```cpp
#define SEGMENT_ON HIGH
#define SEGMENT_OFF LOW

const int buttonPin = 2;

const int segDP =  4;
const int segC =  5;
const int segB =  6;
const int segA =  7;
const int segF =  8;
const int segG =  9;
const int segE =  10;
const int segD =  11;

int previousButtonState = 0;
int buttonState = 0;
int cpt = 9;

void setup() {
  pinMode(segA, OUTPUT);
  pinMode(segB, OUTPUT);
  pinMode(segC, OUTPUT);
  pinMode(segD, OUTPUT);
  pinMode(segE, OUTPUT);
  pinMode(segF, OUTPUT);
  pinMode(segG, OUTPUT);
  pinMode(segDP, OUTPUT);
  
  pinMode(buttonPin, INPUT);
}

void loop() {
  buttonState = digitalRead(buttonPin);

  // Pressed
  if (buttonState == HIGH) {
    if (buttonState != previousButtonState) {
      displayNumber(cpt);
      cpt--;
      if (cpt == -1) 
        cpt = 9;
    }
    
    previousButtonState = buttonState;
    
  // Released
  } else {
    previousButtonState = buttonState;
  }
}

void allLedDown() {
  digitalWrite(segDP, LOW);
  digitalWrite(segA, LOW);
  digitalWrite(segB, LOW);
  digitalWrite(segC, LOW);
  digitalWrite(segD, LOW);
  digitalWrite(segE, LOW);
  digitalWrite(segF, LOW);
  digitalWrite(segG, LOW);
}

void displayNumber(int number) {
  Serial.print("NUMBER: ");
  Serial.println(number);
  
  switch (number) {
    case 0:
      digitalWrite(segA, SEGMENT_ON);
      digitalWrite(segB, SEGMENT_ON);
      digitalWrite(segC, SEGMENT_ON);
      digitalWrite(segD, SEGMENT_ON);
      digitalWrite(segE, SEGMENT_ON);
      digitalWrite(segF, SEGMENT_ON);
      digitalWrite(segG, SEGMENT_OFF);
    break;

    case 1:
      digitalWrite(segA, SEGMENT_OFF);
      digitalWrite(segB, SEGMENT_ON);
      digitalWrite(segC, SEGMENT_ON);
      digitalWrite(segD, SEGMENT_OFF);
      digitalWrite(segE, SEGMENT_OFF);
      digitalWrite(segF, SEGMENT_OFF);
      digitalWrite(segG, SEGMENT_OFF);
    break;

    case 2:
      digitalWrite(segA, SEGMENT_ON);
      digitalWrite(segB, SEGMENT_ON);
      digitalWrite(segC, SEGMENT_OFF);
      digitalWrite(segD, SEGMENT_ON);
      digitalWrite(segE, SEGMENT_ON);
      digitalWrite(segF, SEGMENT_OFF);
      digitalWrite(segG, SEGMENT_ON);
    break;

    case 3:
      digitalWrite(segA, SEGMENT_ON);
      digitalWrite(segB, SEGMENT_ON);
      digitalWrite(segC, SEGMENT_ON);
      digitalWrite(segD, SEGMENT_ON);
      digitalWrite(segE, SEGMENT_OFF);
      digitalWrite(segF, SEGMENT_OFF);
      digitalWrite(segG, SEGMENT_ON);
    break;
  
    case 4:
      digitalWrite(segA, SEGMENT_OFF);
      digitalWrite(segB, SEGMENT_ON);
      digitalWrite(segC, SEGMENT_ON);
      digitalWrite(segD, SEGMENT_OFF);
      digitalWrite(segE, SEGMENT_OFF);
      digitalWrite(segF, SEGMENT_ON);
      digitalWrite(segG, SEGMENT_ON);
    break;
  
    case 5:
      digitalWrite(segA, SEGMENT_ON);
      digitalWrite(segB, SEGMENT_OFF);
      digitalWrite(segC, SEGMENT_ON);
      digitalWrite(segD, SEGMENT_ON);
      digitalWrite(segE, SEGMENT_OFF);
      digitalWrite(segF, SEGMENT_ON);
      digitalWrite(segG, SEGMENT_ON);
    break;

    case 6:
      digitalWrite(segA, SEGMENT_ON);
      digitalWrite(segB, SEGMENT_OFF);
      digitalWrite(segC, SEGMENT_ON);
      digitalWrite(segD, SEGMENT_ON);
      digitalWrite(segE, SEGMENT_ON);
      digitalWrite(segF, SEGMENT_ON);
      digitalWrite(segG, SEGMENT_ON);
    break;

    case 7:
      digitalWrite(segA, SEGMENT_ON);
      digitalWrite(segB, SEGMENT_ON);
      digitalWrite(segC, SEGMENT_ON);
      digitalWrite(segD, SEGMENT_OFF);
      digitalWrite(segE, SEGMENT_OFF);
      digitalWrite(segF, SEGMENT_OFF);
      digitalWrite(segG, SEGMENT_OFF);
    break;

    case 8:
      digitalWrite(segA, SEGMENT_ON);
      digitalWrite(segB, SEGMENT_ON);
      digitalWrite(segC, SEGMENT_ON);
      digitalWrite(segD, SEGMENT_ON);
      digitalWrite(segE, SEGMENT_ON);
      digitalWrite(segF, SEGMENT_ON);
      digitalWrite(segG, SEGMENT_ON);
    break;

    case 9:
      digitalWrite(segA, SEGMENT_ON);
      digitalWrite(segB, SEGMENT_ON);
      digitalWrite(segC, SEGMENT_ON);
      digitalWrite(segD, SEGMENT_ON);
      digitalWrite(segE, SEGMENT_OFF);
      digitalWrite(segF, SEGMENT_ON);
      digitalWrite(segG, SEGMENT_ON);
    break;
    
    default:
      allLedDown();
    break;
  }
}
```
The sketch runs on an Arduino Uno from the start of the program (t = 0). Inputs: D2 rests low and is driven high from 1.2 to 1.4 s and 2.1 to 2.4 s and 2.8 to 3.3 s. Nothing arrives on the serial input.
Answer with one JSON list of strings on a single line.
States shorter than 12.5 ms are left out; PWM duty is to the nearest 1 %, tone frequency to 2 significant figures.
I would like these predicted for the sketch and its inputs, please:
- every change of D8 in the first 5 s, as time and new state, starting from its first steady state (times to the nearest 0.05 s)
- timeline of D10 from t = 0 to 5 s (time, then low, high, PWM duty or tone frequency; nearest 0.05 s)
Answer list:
["0 s low; 1.2 s high; 2.8 s low", "0 s low; 2.1 s high; 2.8 s low"]
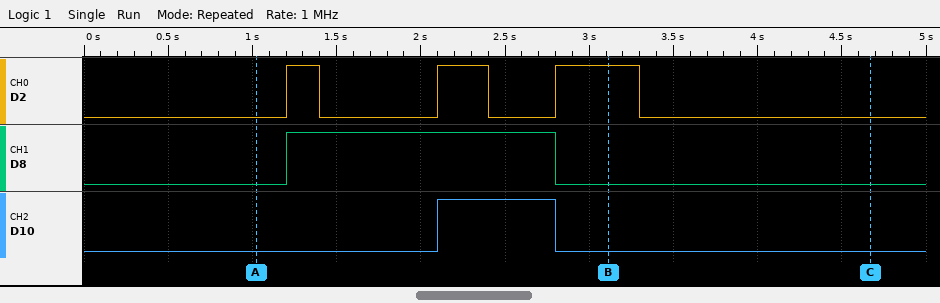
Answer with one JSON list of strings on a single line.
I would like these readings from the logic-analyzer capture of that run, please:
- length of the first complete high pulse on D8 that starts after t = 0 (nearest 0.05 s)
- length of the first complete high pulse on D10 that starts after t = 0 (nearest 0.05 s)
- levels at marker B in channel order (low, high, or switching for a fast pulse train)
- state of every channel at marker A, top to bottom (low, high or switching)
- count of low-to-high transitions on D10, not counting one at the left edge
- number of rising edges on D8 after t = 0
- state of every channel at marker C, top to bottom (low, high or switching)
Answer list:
["1.60 s", "0.70 s", "D2 high, D8 low, D10 low", "D2 low, D8 low, D10 low", "1", "1", "D2 low, D8 low, D10 low"]
